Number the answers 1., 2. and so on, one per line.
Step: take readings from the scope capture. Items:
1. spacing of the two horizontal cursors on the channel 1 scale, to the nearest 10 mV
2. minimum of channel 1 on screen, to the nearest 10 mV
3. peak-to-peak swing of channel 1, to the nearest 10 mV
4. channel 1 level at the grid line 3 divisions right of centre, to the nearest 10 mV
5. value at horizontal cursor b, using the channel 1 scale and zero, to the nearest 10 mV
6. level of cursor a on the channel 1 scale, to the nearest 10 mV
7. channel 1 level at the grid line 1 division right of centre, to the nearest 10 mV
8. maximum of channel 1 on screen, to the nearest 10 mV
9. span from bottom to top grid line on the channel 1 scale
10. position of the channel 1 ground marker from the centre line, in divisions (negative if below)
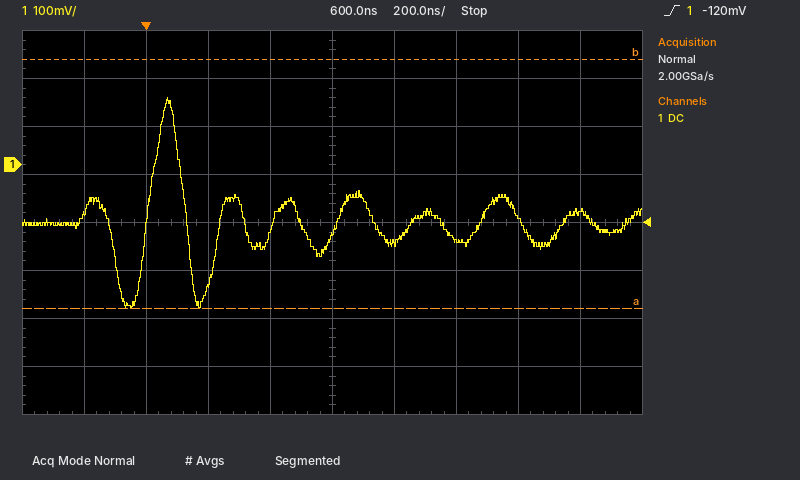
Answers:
1. 520 mV
2. -300 mV
3. 440 mV
4. -110 mV
5. 220 mV
6. -300 mV
7. -160 mV
8. 140 mV
9. 800 mV
10. +1.2 div
